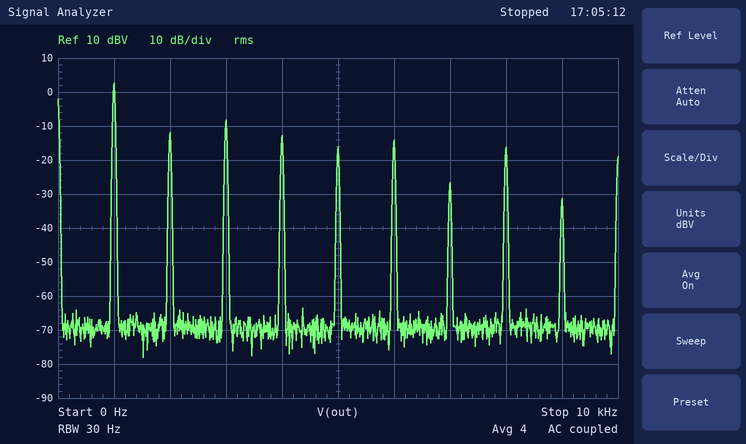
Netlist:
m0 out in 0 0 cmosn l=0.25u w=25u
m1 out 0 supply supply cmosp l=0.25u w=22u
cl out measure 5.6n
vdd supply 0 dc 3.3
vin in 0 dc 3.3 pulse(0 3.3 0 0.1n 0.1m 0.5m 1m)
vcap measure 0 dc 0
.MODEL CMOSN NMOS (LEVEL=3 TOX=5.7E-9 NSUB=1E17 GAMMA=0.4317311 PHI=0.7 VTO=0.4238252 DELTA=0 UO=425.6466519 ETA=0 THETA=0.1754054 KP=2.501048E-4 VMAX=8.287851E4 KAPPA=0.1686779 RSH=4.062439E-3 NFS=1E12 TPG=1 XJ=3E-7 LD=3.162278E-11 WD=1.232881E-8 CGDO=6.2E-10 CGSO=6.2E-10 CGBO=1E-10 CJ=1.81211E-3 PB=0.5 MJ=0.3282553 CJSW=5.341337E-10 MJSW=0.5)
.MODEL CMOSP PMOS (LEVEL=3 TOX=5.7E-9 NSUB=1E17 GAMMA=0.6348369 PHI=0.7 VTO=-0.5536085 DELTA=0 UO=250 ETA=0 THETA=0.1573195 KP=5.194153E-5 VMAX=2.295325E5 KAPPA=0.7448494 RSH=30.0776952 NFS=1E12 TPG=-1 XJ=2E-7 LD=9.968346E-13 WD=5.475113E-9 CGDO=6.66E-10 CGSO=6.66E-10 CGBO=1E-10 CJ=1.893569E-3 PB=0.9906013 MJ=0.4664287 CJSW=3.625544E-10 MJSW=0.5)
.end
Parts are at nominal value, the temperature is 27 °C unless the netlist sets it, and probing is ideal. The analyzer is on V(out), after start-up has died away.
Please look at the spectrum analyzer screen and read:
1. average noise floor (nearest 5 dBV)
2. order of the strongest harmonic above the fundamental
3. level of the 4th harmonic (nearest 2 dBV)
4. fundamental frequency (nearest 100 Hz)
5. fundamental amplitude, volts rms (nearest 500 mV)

-70 dBV
3
-12 dBV
1.0 kHz
1.5 V
